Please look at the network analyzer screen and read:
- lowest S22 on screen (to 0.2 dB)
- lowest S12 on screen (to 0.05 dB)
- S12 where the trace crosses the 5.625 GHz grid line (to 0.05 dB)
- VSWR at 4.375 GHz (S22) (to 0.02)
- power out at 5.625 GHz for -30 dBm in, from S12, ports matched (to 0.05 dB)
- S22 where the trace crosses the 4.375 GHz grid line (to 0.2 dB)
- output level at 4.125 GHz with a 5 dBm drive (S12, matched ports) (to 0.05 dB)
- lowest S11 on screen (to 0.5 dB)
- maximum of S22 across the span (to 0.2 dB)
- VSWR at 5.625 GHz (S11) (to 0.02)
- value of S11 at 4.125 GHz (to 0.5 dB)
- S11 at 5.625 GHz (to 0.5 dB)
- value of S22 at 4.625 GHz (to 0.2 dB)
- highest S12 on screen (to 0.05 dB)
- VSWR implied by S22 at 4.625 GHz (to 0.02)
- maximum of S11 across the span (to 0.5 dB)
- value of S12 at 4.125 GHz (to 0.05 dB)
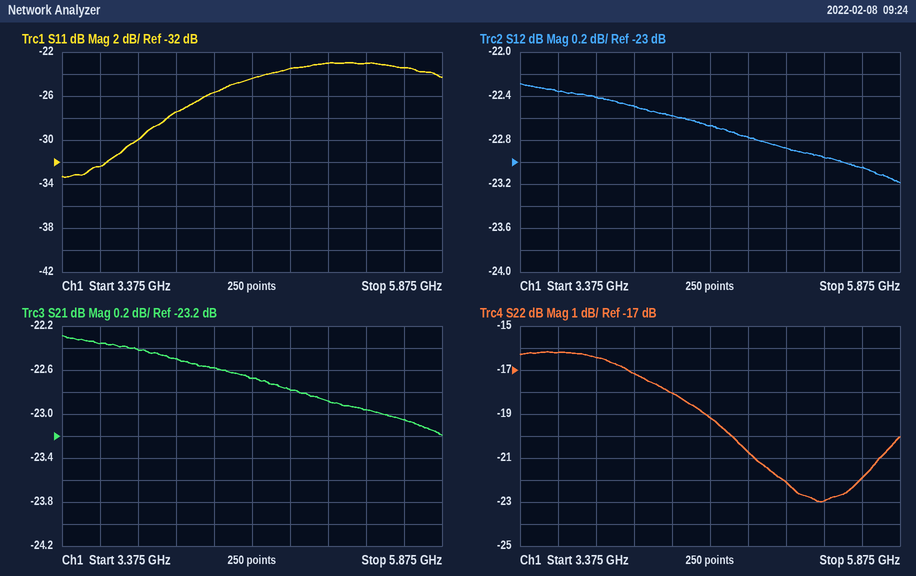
-23.0 dB
-23.20 dB
-23.05 dB
1.28
-53.05 dBm
-18.0 dB
-17.50 dBm
-33.5 dB
-16.2 dB
1.14
-27.5 dB
-23.5 dB
-19.2 dB
-22.30 dB
1.24
-23.0 dB
-22.50 dB
